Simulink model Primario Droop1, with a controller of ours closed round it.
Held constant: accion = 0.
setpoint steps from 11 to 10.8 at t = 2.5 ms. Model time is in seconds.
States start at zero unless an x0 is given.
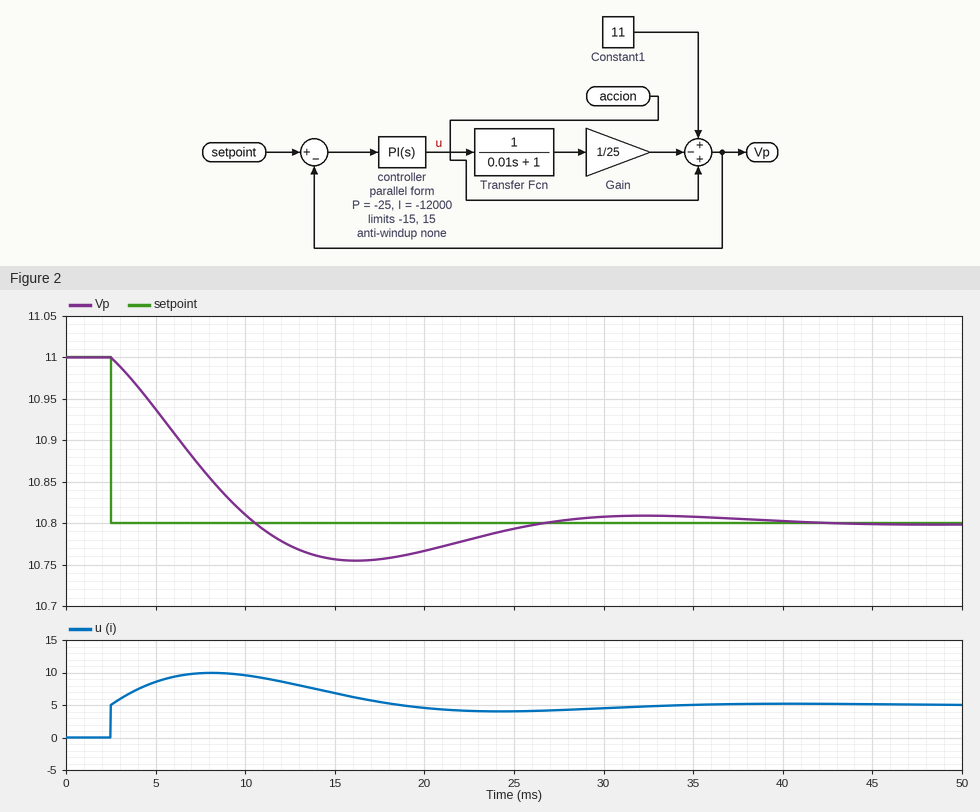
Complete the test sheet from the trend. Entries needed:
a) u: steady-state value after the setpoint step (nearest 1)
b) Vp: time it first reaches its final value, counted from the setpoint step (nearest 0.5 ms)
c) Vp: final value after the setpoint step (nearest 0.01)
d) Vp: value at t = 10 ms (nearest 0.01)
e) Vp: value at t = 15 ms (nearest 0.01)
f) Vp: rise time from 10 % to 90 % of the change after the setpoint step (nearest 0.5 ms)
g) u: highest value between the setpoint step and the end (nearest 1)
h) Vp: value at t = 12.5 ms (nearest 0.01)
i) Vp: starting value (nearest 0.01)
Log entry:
5
8.0 ms
10.80
10.81
10.76
6.0 ms
10
10.77
11.00
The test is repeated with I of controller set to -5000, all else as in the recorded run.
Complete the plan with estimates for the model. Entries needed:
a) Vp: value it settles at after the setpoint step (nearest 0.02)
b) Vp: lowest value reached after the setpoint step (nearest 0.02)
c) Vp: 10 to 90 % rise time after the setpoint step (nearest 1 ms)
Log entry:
10.80
10.78
11 ms
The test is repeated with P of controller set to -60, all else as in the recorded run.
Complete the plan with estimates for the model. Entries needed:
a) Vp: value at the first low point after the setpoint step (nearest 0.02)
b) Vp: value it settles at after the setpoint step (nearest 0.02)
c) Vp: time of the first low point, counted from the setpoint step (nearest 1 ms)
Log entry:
10.78
10.80
13 ms
